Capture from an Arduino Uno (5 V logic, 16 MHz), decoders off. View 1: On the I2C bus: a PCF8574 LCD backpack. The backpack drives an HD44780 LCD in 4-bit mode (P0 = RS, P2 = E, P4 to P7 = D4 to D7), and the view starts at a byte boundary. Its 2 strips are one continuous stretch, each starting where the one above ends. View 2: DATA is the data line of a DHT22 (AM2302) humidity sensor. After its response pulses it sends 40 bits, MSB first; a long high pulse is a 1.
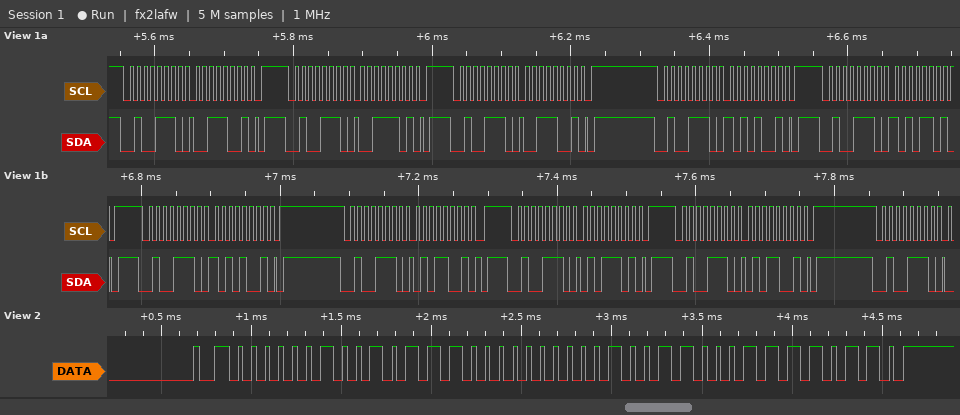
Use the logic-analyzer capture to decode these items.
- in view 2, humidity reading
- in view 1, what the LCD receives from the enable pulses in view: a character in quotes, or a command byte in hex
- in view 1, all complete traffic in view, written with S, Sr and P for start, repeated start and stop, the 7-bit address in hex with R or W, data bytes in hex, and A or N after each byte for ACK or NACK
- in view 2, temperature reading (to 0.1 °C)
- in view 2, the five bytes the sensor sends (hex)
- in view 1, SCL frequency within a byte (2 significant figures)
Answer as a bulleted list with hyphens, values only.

- 60.4 %
- ':'
- S 27W A 39 A P S 27W A 3D A P S 27W A 39 A P S 27W A A9 A P S 27W A AD A P S 27W A A9 A P S 27W A 59 A P S 27W A 5D A P S 27W A 59 A P S 27W A
- 15.2 °C
- 02 5C 00 98 F6
- 100 kHz
